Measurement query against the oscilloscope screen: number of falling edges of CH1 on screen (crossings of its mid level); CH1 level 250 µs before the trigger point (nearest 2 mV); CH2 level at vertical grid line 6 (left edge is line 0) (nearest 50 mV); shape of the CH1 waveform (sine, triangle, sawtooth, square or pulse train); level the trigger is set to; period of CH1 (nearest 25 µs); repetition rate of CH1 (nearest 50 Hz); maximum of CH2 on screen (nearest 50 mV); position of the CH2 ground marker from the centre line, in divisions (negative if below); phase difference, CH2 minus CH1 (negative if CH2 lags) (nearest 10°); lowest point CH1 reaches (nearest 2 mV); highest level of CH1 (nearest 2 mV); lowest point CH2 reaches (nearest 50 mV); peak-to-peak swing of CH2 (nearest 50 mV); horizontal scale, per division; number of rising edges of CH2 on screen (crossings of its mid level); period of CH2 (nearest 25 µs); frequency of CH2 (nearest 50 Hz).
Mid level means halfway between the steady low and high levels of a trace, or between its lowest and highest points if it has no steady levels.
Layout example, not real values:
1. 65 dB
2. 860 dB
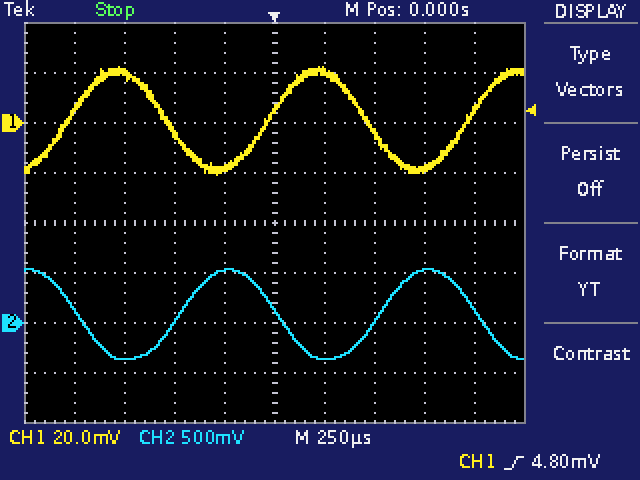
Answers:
1. 2
2. -18 mV
3. -350 mV
4. sine
5. 4.80 mV
6. 1.000 ms
7. 1.00 kHz
8. 550 mV
9. -2.0 div
10. +160°
11. -20 mV
12. 22 mV
13. -350 mV
14. 900 mV
15. 250 µs
16. 2
17. 1.000 ms
18. 1.00 kHz
